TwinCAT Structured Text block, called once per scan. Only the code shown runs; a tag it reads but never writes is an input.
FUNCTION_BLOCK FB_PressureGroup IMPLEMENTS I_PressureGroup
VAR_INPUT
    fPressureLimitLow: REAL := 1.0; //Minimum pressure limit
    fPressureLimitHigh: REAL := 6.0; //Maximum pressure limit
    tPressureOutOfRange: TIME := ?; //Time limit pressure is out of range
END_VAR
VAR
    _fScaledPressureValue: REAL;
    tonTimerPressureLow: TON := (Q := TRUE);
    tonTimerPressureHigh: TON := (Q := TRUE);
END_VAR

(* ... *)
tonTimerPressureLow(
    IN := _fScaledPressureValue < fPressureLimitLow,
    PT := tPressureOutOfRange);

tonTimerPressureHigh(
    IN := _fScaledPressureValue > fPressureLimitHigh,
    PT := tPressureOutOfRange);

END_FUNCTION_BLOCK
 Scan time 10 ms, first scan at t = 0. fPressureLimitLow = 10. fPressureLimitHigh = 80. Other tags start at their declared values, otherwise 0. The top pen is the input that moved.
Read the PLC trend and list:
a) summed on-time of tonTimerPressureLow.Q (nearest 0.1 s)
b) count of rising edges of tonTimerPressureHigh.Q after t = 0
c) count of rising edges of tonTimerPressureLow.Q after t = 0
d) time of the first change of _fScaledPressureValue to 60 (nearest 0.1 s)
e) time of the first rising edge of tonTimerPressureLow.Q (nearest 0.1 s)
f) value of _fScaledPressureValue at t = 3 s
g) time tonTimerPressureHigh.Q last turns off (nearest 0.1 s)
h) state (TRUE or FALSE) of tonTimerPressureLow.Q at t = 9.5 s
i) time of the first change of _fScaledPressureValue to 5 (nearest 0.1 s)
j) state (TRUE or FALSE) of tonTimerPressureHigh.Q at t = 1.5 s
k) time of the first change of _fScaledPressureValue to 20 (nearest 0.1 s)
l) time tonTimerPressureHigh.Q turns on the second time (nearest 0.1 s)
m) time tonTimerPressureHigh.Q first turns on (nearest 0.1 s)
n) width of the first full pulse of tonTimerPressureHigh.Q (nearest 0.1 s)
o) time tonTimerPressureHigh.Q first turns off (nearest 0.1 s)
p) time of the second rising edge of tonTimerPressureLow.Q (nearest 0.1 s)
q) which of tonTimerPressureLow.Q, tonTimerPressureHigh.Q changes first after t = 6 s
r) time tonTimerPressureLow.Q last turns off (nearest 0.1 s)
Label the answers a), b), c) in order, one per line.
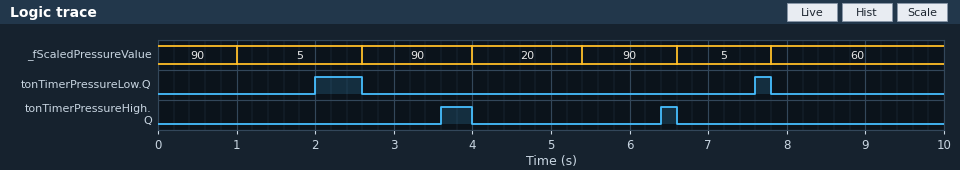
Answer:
a) 0.8 s
b) 2
c) 2
d) 7.8 s
e) 2.0 s
f) 90
g) 6.6 s
h) FALSE
i) 1.0 s
j) FALSE
k) 4.0 s
l) 6.4 s
m) 3.6 s
n) 0.4 s
o) 4.0 s
p) 7.6 s
q) tonTimerPressureHigh.Q
r) 7.8 s
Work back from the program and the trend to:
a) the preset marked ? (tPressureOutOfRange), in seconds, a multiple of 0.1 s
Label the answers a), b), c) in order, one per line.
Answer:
a) 1.0 s
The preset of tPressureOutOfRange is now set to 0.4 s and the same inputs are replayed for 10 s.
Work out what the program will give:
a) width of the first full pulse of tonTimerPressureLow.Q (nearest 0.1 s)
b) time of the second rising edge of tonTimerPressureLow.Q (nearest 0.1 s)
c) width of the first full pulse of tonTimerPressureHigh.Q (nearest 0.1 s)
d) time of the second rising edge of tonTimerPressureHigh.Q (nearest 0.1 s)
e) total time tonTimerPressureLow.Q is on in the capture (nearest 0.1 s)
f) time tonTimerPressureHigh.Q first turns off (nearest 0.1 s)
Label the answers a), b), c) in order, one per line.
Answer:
a) 1.2 s
b) 7.0 s
c) 0.6 s
d) 3.0 s
e) 2.0 s
f) 1.0 s
